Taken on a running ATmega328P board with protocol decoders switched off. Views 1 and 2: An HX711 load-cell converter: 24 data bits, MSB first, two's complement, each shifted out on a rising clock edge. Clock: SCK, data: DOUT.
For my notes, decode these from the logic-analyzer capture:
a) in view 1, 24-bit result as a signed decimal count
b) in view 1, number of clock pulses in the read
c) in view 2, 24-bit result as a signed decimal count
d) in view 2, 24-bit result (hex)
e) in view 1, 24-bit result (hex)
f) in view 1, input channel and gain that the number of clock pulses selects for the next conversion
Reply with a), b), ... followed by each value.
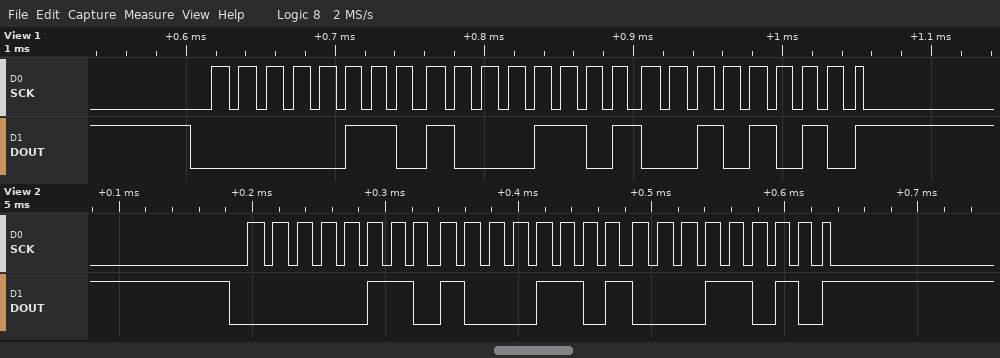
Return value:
a) 429354
b) 25
c) 429338
d) 0x068D1A
e) 0x068D2A
f) channel A, gain 128
